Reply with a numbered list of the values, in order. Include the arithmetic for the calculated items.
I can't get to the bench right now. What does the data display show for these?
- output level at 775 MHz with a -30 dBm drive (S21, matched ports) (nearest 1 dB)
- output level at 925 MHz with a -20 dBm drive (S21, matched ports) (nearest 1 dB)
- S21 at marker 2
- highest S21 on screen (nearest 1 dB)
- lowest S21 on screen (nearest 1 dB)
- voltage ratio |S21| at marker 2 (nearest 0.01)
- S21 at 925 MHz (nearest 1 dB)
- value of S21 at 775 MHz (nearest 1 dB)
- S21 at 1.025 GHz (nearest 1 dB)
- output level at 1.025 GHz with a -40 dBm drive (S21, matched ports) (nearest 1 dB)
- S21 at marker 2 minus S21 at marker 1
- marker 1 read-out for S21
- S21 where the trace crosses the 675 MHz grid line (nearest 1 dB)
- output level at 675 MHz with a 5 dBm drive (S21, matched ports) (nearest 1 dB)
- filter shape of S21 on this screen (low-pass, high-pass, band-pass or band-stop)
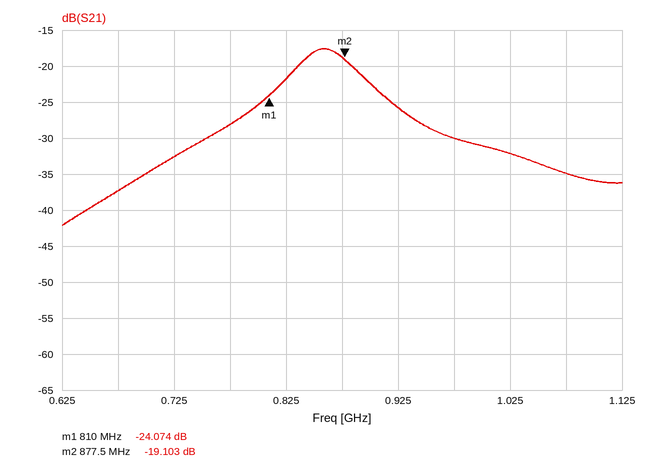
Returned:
1. -30 dBm + (-28 dB) = -58 dBm
2. -20 dBm + (-26 dB) = -46 dBm
3. -19.103 dB
4. -18 dB
5. -42 dB
6. 10^(-19.103/20) ≈ 0.11
7. -26 dB
8. -28 dB
9. -32 dB
10. -40 dBm + (-32 dB) = -72 dBm
11. -19.103 − (-24.074) = 4.971 dB
12. -24.074 dB
13. -37 dB
14. 5 dBm + (-37 dB) = -32 dBm
15. band-pass
